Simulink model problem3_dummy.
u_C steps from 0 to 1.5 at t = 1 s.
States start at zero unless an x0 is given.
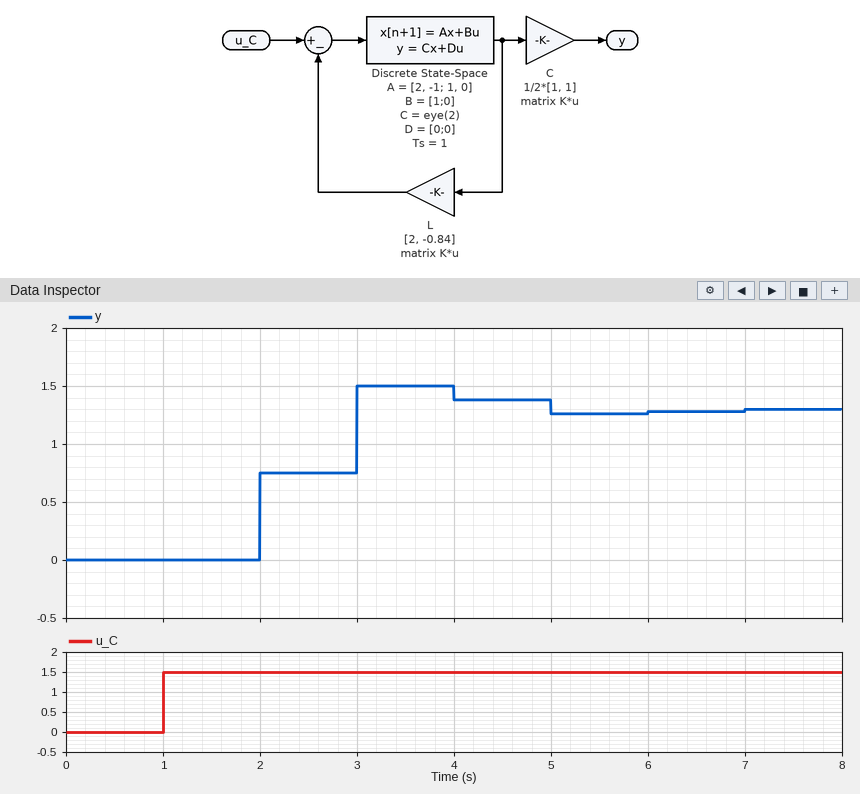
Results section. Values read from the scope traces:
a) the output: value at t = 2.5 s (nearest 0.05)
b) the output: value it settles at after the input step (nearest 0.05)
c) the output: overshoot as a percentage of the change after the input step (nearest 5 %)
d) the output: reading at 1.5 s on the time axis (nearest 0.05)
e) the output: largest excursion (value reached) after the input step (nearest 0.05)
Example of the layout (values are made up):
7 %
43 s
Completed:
0.75
1.30
15 %
0.00
1.50
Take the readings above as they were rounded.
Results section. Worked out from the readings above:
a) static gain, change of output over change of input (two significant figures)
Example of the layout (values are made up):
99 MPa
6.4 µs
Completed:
0.87
